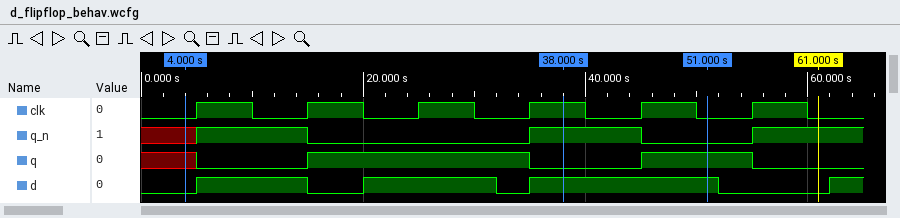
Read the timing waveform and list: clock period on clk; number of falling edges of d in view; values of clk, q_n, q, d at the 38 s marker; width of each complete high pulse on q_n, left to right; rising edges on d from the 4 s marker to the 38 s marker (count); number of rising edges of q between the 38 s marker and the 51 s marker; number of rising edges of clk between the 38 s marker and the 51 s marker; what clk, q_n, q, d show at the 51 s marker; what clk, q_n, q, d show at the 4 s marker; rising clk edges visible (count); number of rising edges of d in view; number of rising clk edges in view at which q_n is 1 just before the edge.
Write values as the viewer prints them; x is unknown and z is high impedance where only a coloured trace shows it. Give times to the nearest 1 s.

10 s
3
clk=1, q_n=1, q=0, d=1
10 s
3
1
1
clk=0, q_n=0, q=1, d=1
clk=0, q_n=x, q=x, d=0
6
4
2
